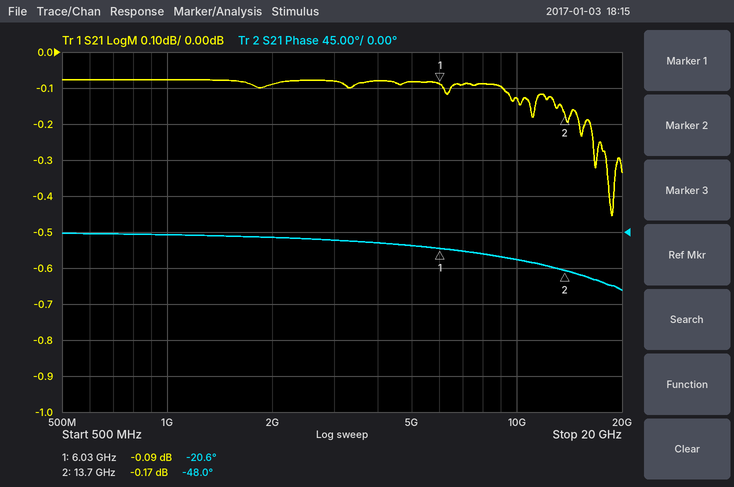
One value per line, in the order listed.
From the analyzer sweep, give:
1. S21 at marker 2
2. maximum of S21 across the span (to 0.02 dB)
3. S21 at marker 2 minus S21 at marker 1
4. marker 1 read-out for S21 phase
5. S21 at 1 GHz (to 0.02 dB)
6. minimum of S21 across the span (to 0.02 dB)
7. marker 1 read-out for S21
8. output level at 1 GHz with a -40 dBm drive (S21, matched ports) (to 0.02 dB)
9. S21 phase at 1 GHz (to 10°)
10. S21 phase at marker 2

-0.17 dB
-0.08 dB
-0.08 dB
-20.6°
-0.08 dB
-0.46 dB
-0.09 dB
-40.08 dBm
0°
-48.0°
